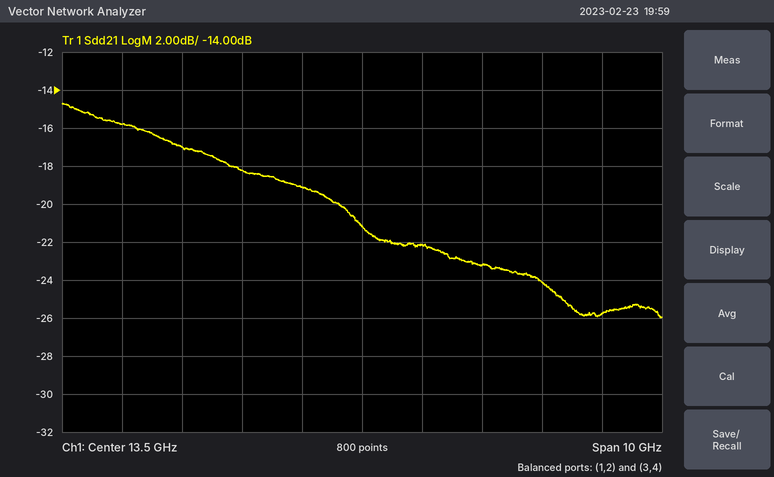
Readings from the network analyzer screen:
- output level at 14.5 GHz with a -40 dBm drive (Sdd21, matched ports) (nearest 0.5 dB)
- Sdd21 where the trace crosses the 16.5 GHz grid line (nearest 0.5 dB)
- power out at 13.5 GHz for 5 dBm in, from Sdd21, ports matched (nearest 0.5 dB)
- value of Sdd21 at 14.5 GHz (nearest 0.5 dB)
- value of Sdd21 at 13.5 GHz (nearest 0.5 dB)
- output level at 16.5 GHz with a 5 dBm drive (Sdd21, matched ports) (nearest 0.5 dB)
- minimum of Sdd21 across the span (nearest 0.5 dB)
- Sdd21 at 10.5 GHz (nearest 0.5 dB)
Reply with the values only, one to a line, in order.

-62.0 dBm
-24.0 dB
-16.0 dBm
-22.0 dB
-21.0 dB
-19.0 dBm
-26.0 dB
-17.0 dB
